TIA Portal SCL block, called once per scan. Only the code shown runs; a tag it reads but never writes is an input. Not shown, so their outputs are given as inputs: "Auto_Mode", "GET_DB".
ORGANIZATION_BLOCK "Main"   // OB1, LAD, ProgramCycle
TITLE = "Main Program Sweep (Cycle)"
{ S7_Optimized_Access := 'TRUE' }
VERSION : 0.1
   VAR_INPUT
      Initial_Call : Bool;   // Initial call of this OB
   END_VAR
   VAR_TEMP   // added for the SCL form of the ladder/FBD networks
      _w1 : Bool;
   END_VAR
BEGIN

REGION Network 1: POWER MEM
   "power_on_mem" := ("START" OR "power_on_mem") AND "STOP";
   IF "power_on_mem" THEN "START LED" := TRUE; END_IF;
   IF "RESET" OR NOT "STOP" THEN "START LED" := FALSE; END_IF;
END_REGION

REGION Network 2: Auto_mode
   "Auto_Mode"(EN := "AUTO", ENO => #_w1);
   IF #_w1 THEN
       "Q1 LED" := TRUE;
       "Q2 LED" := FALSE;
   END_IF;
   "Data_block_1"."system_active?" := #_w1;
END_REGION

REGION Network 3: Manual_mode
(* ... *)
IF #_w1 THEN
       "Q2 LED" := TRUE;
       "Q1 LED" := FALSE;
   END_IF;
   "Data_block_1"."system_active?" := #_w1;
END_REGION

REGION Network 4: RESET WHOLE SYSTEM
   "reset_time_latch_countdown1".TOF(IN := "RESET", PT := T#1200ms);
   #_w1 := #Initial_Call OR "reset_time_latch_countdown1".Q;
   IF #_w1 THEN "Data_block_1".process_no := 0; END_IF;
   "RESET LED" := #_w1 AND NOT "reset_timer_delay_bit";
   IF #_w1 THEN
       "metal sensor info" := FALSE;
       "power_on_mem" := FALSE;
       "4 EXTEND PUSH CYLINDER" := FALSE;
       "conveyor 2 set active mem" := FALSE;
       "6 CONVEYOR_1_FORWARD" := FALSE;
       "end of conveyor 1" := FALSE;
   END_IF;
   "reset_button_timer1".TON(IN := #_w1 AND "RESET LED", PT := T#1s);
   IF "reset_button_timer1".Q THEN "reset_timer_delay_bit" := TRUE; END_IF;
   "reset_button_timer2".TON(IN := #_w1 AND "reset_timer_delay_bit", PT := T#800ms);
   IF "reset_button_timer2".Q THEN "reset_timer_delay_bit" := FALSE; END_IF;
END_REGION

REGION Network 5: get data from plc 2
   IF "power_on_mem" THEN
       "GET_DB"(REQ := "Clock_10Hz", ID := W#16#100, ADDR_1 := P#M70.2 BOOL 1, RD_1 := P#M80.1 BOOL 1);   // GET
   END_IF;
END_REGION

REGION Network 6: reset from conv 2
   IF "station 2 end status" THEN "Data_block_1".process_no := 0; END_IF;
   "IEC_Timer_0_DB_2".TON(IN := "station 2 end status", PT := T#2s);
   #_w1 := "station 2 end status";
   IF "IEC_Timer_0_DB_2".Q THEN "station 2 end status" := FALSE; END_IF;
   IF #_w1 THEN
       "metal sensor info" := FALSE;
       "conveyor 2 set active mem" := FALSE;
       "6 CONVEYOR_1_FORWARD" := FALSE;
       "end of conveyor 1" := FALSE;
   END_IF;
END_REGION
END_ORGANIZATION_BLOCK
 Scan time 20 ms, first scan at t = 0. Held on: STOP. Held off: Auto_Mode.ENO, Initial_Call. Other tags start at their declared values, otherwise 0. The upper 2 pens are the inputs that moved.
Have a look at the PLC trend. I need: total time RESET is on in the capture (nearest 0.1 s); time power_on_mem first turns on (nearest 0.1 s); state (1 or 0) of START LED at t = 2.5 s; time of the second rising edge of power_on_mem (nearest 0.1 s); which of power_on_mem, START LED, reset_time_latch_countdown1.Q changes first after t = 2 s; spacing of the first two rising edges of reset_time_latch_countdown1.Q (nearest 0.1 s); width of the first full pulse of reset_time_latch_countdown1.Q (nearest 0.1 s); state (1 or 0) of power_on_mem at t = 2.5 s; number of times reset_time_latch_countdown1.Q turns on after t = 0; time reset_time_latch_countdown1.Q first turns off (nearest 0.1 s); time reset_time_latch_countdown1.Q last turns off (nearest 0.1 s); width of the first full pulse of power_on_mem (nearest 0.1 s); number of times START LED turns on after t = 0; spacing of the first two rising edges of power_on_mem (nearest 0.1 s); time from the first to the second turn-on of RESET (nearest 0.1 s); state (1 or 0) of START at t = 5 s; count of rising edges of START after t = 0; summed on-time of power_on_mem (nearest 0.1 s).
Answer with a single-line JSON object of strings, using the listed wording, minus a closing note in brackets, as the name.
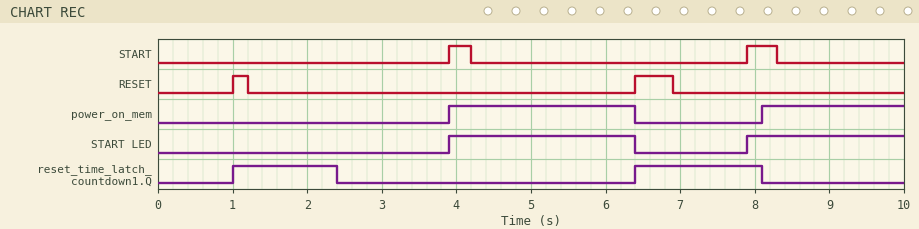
{"total time RESET is on in the capture": "0.7 s", "time power_on_mem first turns on": "3.9 s", "state (1 or 0) of START LED at t = 2.5 s": "0", "time of the second rising edge of power_on_mem": "8.1 s", "which of power_on_mem, START LED, reset_time_latch_countdown1.Q changes first after t = 2 s": "reset_time_latch_countdown1.Q", "spacing of the first two rising edges of reset_time_latch_countdown1.Q": "5.4 s", "width of the first full pulse of reset_time_latch_countdown1.Q": "1.4 s", "state (1 or 0) of power_on_mem at t = 2.5 s": "0", "number of times reset_time_latch_countdown1.Q turns on after t = 0": "2", "time reset_time_latch_countdown1.Q first turns off": "2.4 s", "time reset_time_latch_countdown1.Q last turns off": "8.1 s", "width of the first full pulse of power_on_mem": "2.5 s", "number of times START LED turns on after t = 0": "2", "spacing of the first two rising edges of power_on_mem": "4.2 s", "time from the first to the second turn-on of RESET": "5.4 s", "state (1 or 0) of START at t = 5 s": "0", "count of rising edges of START after t = 0": "2", "summed on-time of power_on_mem": "4.4 s"}
